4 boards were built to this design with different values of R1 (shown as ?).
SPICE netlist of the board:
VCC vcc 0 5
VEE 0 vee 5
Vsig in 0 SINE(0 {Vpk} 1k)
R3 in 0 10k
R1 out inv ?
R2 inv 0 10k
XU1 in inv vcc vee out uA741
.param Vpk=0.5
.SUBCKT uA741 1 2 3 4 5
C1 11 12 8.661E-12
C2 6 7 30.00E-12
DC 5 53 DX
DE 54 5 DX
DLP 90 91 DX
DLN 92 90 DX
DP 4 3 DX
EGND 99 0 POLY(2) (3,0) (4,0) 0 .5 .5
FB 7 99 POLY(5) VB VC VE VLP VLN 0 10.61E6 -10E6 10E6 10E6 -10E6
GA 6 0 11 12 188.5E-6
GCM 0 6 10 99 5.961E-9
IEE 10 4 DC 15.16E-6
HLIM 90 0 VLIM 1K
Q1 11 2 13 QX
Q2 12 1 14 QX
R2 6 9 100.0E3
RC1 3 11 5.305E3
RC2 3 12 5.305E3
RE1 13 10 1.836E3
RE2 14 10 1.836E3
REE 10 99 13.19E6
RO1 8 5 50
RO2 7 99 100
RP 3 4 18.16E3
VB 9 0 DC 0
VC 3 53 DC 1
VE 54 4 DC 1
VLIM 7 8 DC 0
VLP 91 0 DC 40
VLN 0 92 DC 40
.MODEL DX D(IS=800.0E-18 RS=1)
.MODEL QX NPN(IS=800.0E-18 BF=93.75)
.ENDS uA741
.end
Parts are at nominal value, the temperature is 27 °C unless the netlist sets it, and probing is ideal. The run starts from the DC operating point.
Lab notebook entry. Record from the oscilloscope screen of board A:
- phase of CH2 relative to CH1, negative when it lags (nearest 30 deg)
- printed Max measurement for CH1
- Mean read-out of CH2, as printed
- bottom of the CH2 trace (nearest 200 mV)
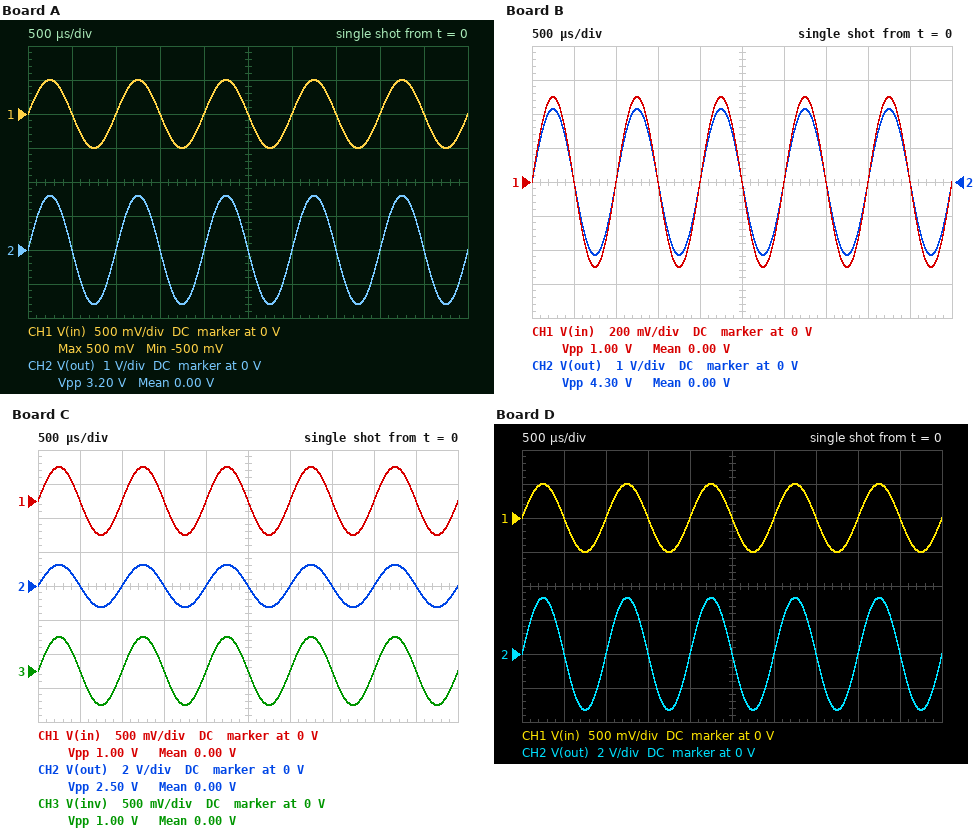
0 deg
500 mV
0.00 V
-1.6 V
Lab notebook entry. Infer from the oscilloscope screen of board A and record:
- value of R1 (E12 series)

22 kΩ
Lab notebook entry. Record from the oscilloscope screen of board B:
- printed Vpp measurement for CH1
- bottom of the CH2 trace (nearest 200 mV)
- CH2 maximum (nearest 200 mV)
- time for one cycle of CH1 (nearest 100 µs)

1.00 V
-2.2 V
2.2 V
1.0 ms
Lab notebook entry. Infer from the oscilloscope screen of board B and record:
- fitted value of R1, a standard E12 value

33 kΩ
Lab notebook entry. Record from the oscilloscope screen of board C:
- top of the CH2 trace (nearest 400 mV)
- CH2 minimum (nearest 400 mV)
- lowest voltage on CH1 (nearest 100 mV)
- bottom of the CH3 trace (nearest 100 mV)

1.2 V
-1.2 V
-500 mV
-500 mV
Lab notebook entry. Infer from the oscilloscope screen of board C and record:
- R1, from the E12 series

15 kΩ
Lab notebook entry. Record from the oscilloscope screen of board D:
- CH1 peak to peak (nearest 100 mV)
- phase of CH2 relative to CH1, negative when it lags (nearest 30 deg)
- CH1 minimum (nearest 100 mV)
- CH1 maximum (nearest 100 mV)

1.0 V
0 deg
-500 mV
500 mV
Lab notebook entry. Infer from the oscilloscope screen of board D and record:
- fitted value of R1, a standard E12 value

56 kΩ
